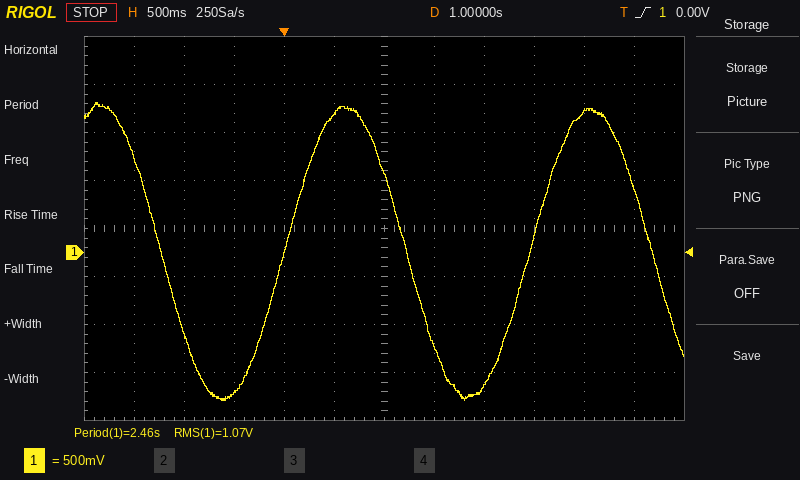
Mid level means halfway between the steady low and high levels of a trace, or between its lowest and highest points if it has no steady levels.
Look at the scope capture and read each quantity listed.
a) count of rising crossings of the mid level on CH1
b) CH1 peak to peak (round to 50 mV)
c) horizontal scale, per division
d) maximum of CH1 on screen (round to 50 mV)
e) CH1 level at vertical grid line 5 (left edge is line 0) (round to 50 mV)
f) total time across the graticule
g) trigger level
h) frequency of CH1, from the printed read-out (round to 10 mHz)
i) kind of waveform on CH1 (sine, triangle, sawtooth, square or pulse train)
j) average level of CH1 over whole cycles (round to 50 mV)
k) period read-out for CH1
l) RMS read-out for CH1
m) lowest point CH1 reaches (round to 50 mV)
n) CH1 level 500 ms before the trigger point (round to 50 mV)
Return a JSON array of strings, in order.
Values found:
["2", "3.10 V", "500 ms", "1.55 V", "1.45 V", "6 s", "0.00 V", "410 mHz", "sine", "0 mV", "2.46 s", "1.07 V", "-1.55 V", "-1.45 V"]
